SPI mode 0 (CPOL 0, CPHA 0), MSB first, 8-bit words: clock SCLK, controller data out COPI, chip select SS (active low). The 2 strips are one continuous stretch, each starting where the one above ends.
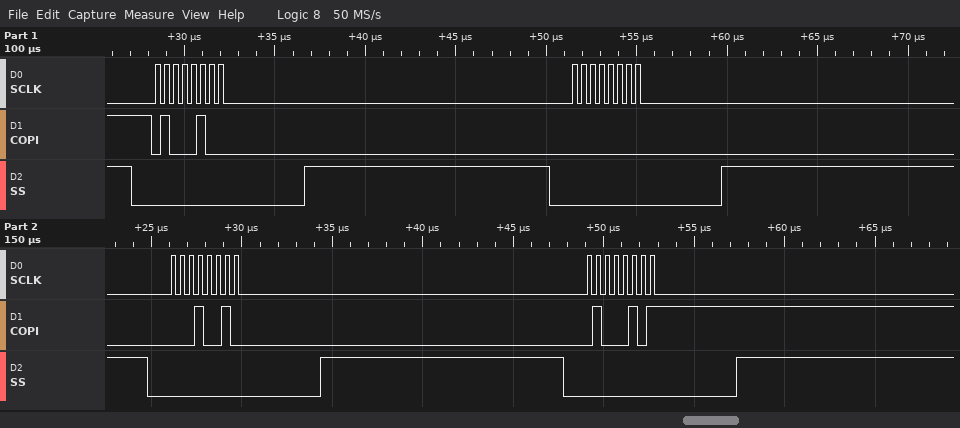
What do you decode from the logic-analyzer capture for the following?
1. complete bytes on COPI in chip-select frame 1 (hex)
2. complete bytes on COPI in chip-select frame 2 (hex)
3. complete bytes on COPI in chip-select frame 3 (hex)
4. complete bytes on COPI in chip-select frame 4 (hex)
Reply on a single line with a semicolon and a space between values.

0x44; 0x00; 0x12; 0x45
